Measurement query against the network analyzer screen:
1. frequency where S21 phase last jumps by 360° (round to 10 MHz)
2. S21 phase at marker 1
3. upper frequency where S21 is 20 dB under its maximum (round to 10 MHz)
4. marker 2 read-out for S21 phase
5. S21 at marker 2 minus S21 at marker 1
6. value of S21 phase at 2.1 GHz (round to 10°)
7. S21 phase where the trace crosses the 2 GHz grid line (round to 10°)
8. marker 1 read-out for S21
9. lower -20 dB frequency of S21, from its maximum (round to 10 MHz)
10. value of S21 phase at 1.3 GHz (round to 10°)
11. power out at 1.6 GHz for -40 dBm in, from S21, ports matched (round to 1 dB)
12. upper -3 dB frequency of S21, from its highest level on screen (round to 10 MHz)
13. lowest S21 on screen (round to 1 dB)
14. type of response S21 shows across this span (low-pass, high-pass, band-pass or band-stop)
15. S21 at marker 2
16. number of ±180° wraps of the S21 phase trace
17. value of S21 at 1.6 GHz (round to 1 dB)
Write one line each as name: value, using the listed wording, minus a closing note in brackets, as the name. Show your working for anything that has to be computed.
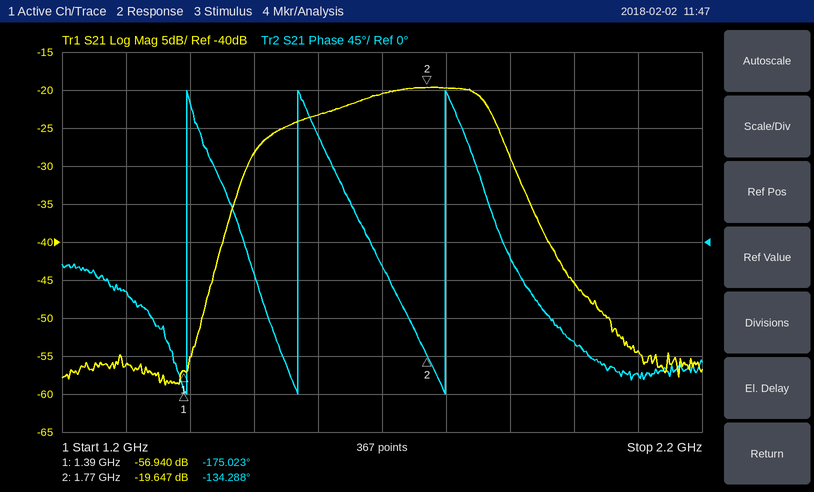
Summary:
frequency where S21 phase last jumps by 360°: 1.80 GHz
S21 phase at marker 1: -175.023°
upper frequency where S21 is 20 dB under its maximum: 1.96 GHz
marker 2 read-out for S21 phase: -134.288°
S21 at marker 2 minus S21 at marker 1: -19.647 − (-56.94) = 37.293 dB
value of S21 phase at 2.1 GHz: -160°
S21 phase where the trace crosses the 2 GHz grid line: -120°
marker 1 read-out for S21: -56.940 dB
lower -20 dB frequency of S21, from its maximum: 1.45 GHz
value of S21 phase at 1.3 GHz: -60°
power out at 1.6 GHz for -40 dBm in, from S21, ports matched: -40 dBm + (-23 dB) = -63 dBm
upper -3 dB frequency of S21, from its highest level on screen: 1.87 GHz
lowest S21 on screen: -59 dB
type of response S21 shows across this span: band-pass
S21 at marker 2: -19.647 dB
number of ±180° wraps of the S21 phase trace: 3
value of S21 at 1.6 GHz: -23 dB
